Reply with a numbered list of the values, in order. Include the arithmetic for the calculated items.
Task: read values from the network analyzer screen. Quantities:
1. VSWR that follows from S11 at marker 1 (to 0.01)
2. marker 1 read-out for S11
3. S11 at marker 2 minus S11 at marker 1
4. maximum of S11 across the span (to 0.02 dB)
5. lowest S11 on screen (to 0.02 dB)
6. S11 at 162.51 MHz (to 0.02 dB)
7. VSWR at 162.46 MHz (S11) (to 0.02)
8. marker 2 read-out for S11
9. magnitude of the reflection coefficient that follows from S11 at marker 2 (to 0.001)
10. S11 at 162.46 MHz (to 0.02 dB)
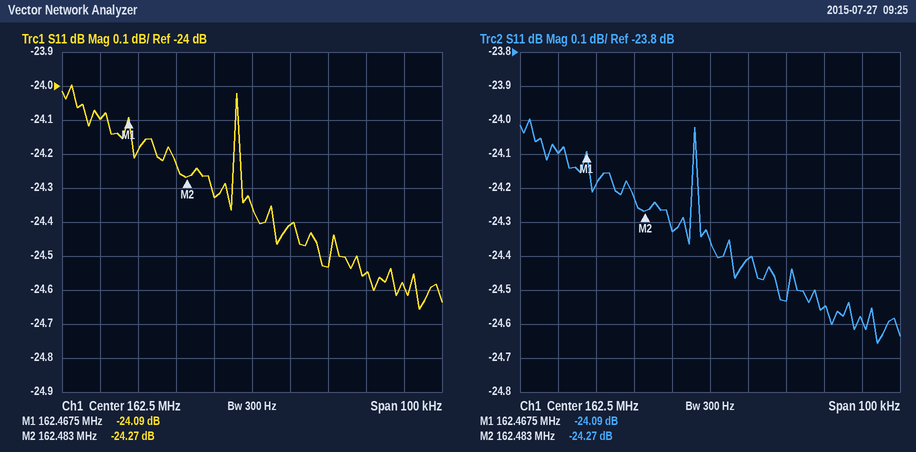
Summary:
1. (1 + 0.0624)/(1 − 0.0624) ≈ 1.13
2. -24.09 dB
3. -24.27 − (-24.09) = -0.18 dB
4. -24.00 dB
5. -24.66 dB
6. -24.40 dB
7. |Γ| = 10^(-24.1/20) = 0.0624; VSWR = (1 + 0.0624)/(1 − 0.0624) ≈ 1.13, so 1.14 to the nearest 0.02
8. -24.27 dB
9. 10^(-24.27/20) ≈ 0.061
10. -24.10 dB
